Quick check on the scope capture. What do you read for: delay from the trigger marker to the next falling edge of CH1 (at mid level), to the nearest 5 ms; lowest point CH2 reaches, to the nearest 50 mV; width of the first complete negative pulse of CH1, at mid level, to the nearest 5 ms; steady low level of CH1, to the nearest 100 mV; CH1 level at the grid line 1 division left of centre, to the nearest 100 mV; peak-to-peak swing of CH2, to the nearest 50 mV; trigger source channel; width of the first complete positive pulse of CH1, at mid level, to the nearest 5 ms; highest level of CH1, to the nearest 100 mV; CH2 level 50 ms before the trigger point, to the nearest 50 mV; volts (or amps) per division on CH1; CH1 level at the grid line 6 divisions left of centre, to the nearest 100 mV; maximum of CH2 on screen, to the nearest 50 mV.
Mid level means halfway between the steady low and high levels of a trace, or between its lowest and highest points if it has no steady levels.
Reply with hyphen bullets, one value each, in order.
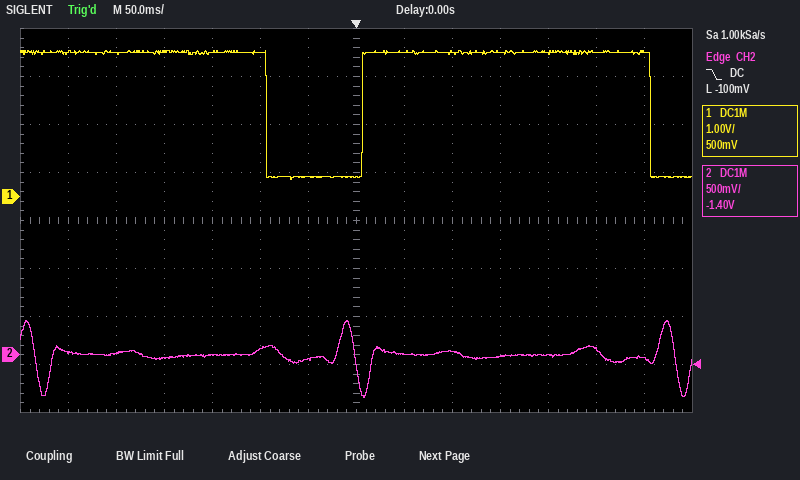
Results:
- 305 ms
- -450 mV
- 100 ms
- 400 mV
- 400 mV
- 800 mV
- CH2
- 300 ms
- 3.0 V
- -50 mV
- 1 V
- 3.0 V
- 350 mV
